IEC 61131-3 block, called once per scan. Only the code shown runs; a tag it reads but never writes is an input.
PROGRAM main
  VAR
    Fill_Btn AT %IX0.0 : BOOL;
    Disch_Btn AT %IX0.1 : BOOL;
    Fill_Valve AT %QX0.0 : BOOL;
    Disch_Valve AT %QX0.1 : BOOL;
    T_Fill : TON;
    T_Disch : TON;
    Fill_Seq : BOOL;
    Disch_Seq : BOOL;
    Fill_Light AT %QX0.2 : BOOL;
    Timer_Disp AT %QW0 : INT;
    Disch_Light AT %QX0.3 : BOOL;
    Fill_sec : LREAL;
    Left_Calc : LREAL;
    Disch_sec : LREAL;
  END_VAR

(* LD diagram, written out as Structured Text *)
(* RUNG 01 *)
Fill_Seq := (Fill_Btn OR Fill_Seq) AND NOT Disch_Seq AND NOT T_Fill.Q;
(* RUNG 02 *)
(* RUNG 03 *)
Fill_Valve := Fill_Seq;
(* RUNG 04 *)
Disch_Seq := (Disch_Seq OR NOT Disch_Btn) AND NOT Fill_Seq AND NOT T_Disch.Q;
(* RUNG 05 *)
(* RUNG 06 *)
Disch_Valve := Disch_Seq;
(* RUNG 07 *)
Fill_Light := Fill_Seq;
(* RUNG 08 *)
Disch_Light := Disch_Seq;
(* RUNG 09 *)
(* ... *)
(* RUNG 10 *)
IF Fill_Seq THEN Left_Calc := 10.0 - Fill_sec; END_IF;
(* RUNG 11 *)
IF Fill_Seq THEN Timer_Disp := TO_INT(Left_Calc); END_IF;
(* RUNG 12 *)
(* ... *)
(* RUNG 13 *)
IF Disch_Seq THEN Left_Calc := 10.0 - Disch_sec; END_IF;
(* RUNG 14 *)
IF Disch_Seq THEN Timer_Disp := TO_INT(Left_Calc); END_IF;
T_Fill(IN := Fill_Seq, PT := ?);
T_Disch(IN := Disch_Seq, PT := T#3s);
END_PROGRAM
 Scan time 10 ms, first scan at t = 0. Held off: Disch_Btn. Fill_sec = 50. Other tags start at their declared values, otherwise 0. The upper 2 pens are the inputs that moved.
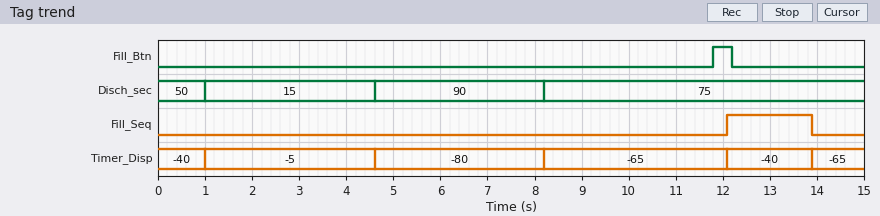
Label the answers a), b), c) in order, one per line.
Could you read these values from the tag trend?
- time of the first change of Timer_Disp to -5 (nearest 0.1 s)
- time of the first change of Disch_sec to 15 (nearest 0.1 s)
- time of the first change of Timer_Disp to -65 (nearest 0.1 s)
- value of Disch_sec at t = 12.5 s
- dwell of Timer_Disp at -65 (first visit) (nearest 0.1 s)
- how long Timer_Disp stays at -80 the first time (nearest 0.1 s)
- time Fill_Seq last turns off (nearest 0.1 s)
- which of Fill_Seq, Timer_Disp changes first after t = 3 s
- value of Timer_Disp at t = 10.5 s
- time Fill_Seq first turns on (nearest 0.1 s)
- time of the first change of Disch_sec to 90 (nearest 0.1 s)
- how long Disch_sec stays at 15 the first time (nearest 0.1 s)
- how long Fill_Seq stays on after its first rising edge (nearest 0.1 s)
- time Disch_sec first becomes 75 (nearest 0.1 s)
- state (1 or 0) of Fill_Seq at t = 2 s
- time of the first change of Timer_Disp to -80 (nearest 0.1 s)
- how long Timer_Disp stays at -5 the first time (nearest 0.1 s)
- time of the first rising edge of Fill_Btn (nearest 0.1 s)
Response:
a) 1.0 s
b) 1.0 s
c) 8.2 s
d) 75
e) 3.9 s
f) 3.6 s
g) 13.9 s
h) Timer_Disp
i) -65
j) 12.1 s
k) 4.6 s
l) 3.6 s
m) 1.8 s
n) 8.2 s
o) 0
p) 4.6 s
q) 3.6 s
r) 11.8 s
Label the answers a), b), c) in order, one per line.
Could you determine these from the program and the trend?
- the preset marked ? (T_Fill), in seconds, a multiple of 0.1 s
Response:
a) 1.8 s
